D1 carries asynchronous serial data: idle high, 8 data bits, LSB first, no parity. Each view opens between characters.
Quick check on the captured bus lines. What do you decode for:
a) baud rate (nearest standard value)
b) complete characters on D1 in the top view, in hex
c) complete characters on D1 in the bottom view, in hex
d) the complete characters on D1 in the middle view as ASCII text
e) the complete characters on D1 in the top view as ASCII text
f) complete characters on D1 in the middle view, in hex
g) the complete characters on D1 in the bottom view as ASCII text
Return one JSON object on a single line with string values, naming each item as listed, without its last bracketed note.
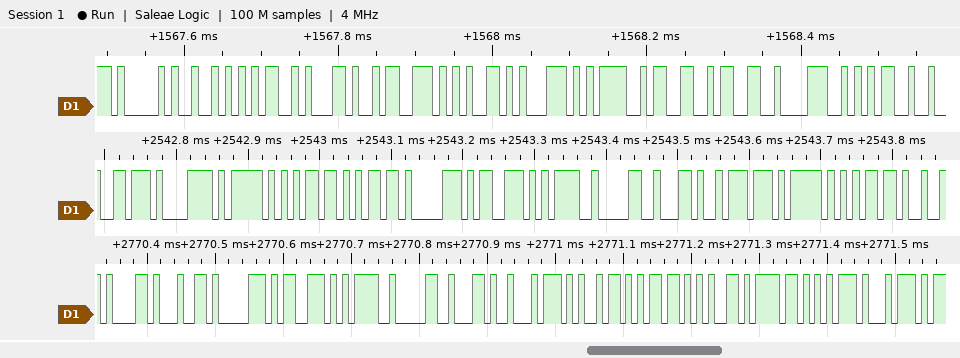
{"baud rate": "115200 baud", "complete characters on D1 in the top view, in hex": "41, 52, 4D, 2C, 73, 65, 71, 3D, 33, 33, 38, 35", "complete characters on D1 in the bottom view, in hex": "61, 64, 70, 73, 3D, 30, 2C, 74, 69, 6D, 65, 6F, 75, 74", "the complete characters on D1 in the middle view as ASCII text": "\"vx_mmps=0,w_m\"", "the complete characters on D1 in the top view as ASCII text": "\"ARM,seq=3385\"", "complete characters on D1 in the middle view, in hex": "76, 78, 5F, 6D, 6D, 70, 73, 3D, 30, 2C, 77, 5F, 6D", "the complete characters on D1 in the bottom view as ASCII text": "\"adps=0,timeout\""}
